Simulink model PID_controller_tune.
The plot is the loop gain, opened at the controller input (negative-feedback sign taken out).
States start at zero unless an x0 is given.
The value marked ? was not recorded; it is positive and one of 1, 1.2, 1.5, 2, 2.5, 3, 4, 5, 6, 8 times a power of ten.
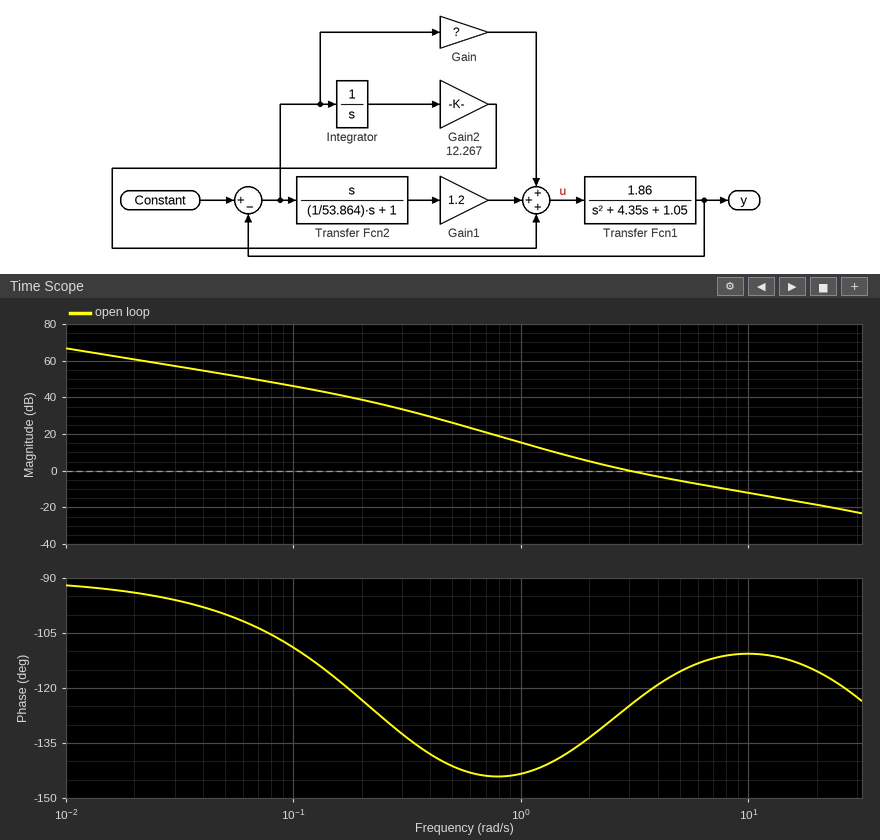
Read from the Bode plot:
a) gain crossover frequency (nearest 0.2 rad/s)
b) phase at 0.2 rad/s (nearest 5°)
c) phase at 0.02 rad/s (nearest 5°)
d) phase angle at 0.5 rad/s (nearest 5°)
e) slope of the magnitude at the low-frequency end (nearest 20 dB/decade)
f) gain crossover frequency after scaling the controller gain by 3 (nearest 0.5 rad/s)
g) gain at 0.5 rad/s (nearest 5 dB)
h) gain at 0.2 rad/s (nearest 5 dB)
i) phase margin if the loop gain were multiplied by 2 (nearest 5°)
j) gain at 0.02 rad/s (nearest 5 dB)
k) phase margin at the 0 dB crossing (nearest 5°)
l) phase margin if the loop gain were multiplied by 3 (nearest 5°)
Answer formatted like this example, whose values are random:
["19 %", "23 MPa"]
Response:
["3.0 rad/s", "-125°", "-95°", "-140°", "-20 dB/decade", "7.5 rad/s", "25 dB", "40 dB", "65°", "60 dB", "55°", "70°"]
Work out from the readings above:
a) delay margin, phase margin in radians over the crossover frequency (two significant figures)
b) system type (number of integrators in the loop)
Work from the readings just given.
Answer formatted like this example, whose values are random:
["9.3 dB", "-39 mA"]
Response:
["0.32 s", "1"]
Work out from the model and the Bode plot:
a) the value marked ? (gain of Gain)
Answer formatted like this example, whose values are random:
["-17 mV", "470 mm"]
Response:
["8"]
